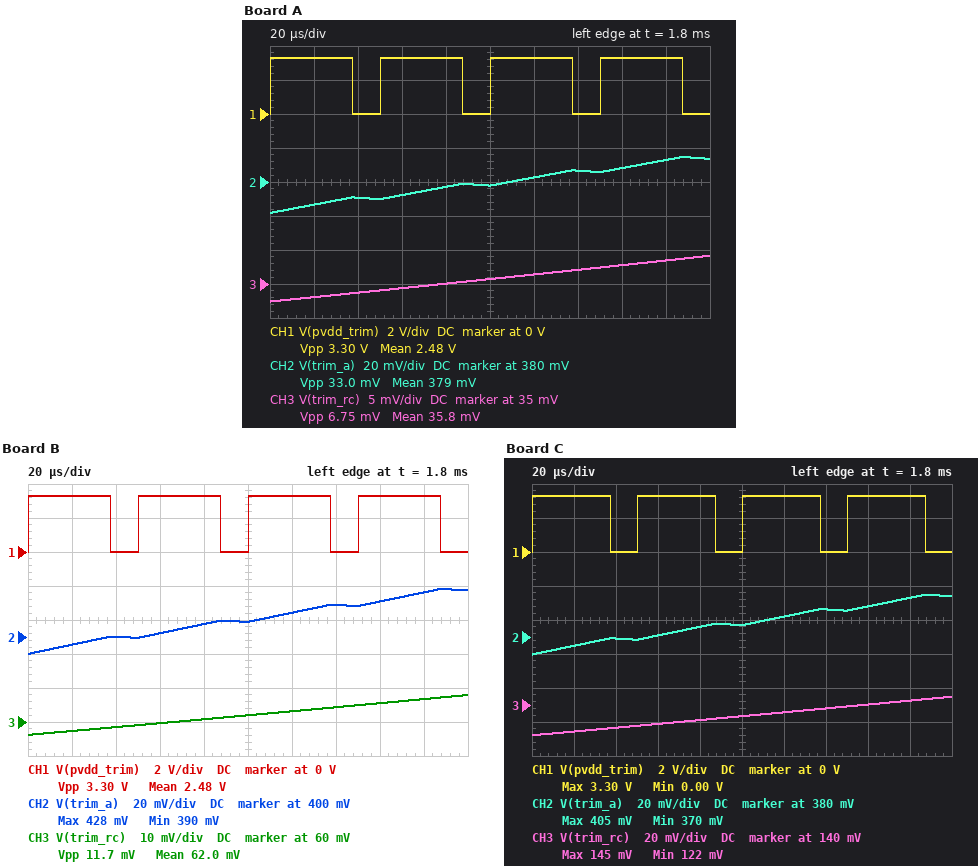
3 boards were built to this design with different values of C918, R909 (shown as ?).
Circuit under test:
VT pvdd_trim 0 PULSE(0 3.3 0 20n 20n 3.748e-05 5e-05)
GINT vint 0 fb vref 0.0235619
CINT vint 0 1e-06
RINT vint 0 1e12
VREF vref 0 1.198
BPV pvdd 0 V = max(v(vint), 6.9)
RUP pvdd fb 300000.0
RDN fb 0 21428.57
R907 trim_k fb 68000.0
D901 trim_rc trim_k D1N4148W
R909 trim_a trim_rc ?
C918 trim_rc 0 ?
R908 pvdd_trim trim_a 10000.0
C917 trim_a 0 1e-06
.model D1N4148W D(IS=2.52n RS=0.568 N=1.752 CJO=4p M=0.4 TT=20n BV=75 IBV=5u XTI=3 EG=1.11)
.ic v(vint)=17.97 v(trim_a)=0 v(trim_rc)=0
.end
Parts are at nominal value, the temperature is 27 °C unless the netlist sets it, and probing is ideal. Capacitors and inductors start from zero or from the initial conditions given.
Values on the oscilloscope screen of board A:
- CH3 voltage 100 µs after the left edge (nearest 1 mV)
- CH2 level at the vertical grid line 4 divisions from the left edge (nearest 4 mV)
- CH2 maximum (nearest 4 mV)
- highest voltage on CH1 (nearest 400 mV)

36 mV
376 mV
396 mV
3.2 V
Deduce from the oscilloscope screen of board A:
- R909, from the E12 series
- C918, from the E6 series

6.8 kΩ
1.5 µF
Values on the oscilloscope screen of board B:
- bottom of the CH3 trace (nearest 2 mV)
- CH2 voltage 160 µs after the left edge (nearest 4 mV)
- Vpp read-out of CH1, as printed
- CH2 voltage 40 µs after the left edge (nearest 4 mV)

56 mV
420 mV
3.30 V
400 mV
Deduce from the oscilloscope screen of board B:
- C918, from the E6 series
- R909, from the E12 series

330 nF
18 kΩ
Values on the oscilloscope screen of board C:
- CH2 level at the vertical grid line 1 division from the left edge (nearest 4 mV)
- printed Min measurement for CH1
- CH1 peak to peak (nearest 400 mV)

376 mV
0.00 V
3.2 V
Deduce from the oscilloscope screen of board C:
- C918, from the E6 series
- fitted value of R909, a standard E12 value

330 nF
6.8 kΩ
